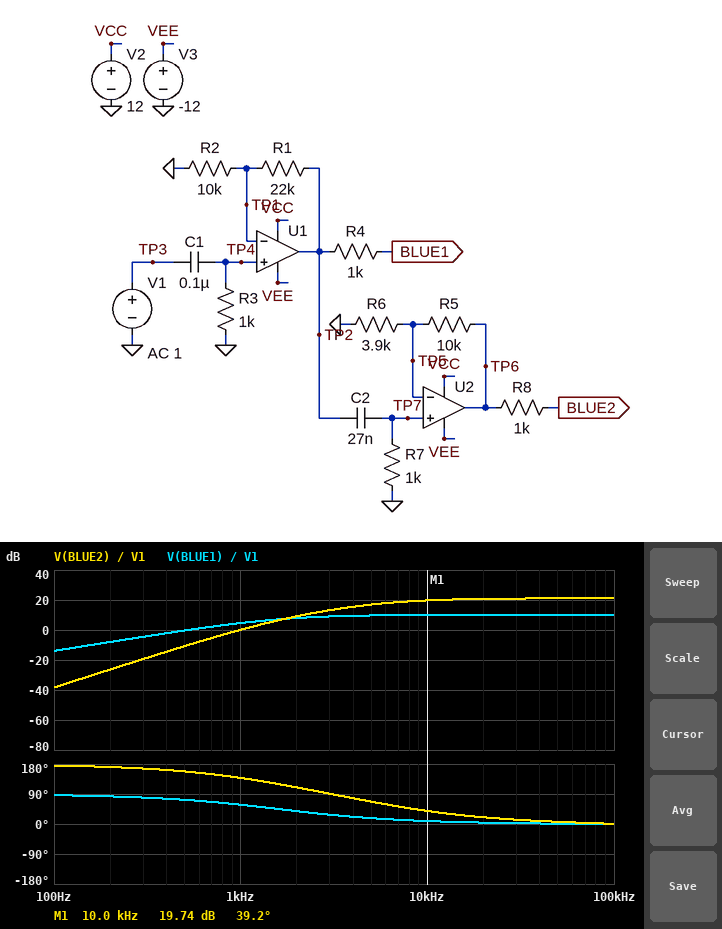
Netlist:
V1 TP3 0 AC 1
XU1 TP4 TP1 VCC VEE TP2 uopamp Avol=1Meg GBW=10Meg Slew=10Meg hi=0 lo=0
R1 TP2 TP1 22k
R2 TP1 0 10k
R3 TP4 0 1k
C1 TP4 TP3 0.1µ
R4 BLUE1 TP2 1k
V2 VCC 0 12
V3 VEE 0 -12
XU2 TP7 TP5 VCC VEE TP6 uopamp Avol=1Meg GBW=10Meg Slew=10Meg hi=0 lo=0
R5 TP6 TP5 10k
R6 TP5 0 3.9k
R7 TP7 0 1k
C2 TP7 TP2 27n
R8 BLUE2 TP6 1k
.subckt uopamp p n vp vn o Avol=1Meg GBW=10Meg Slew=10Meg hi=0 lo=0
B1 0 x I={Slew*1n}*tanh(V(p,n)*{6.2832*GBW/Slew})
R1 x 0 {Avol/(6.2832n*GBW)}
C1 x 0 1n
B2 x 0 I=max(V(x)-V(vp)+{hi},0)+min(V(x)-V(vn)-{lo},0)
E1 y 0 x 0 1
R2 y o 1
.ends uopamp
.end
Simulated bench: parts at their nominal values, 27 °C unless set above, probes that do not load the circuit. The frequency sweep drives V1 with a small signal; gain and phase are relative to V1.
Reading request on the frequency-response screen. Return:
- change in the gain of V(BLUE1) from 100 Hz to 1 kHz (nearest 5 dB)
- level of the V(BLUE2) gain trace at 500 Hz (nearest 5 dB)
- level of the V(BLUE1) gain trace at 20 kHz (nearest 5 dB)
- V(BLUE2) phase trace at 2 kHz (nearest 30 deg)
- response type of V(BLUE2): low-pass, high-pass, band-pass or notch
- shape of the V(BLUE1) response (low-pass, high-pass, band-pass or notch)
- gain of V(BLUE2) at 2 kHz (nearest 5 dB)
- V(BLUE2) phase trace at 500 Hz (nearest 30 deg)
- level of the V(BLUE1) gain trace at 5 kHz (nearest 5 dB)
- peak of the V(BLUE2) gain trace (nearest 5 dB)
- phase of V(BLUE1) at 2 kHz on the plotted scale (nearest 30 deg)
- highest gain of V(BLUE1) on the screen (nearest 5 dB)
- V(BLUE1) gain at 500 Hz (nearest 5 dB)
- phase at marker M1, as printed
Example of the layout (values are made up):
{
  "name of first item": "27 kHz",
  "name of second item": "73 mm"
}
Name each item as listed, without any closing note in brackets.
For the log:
{
  "change in the gain of V(BLUE1) from 100 Hz to 1 kHz": "20 dB",
  "level of the V(BLUE2) gain trace at 500 Hz": "-10 dB",
  "level of the V(BLUE1) gain trace at 20 kHz": "10 dB",
  "V(BLUE2) phase trace at 2 kHz": "120 deg",
  "response type of V(BLUE2): low-pass, high-pass, band-pass or notch": "high-pass",
  "shape of the V(BLUE1) response": "high-pass",
  "gain of V(BLUE2) at 2 kHz": "10 dB",
  "V(BLUE2) phase trace at 500 Hz": "150 deg",
  "level of the V(BLUE1) gain trace at 5 kHz": "10 dB",
  "peak of the V(BLUE2) gain trace": "20 dB",
  "phase of V(BLUE1) at 2 kHz on the plotted scale": "30 deg",
  "highest gain of V(BLUE1) on the screen": "10 dB",
  "V(BLUE1) gain at 500 Hz": "0 dB",
  "phase at marker M1, as printed": "39.2 deg"
}
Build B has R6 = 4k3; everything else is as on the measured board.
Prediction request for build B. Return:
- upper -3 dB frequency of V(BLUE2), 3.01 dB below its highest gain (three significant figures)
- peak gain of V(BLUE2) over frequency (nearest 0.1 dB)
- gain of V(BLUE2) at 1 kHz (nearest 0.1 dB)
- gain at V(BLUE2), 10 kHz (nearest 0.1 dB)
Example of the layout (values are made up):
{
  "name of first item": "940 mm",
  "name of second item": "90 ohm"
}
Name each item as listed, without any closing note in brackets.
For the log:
{
  "upper -3 dB frequency of V(BLUE2), 3.01 dB below its highest gain": "1.98 MHz",
  "peak gain of V(BLUE2) over frequency": "20.5 dB",
  "gain of V(BLUE2) at 1 kHz": "-0.5 dB",
  "gain at V(BLUE2), 10 kHz": "19.1 dB"
}
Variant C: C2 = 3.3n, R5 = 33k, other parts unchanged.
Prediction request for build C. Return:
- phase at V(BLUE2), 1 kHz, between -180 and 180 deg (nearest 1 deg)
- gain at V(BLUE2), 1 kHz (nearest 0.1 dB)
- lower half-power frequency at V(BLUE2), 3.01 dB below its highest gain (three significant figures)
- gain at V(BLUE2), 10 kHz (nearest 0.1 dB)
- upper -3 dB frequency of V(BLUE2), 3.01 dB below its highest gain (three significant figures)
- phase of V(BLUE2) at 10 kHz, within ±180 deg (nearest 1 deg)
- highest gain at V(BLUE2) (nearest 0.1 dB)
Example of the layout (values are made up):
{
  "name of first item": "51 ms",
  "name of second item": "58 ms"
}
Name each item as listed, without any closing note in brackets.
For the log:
{
  "phase at V(BLUE2), 1 kHz, between -180 and 180 deg": "147 deg",
  "gain at V(BLUE2), 1 kHz": "-9.5 dB",
  "lower half-power frequency at V(BLUE2), 3.01 dB below its highest gain": "44.2 kHz",
  "gain at V(BLUE2), 10 kHz": "15.7 dB",
  "upper -3 dB frequency of V(BLUE2), 3.01 dB below its highest gain": "1.04 MHz",
  "phase of V(BLUE2) at 10 kHz, within ±180 deg": "87 deg",
  "highest gain at V(BLUE2)": "29.2 dB"
}
